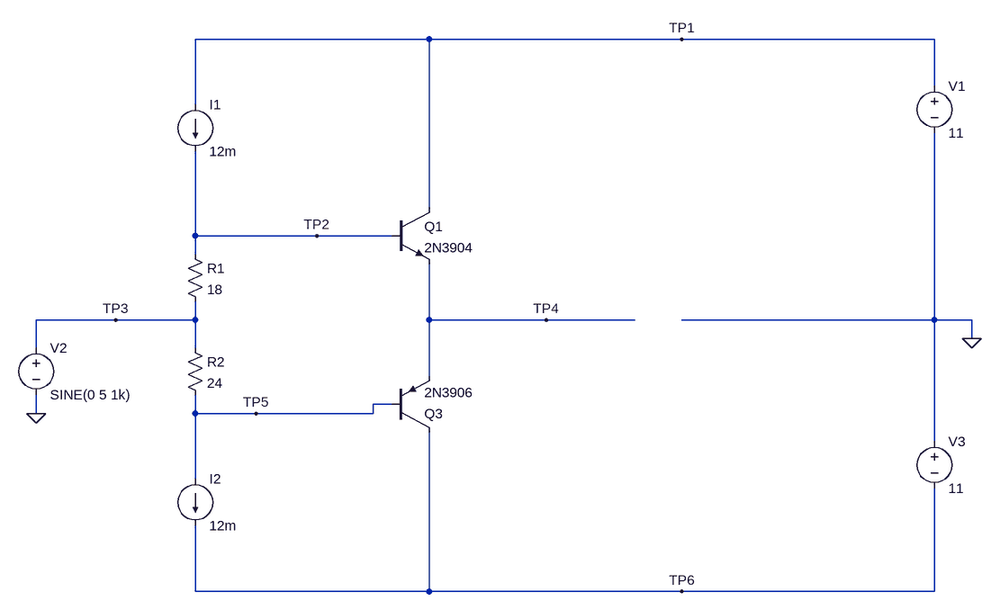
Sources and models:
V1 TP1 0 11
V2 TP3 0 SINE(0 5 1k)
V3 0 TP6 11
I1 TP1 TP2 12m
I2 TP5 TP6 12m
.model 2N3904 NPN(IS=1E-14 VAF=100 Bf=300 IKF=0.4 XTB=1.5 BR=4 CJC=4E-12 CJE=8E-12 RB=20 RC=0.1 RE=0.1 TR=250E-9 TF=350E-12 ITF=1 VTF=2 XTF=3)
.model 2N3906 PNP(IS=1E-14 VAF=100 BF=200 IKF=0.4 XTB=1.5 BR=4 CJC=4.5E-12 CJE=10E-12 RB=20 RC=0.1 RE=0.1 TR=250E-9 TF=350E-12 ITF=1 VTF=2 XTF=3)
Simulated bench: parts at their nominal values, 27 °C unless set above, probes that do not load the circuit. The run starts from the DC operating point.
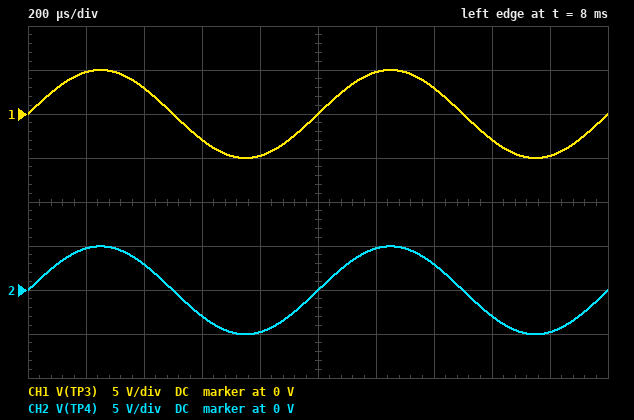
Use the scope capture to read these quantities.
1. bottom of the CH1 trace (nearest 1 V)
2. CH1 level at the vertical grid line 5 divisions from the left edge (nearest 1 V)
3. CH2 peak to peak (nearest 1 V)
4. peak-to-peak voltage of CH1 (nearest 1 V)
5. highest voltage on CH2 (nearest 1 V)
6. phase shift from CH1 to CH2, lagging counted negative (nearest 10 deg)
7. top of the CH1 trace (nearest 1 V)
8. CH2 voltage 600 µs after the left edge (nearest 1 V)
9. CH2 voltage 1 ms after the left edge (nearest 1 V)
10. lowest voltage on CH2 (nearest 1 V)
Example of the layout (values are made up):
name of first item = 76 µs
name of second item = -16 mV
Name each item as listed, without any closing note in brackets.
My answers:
bottom of the CH1 trace = -5 V
CH1 level at the vertical grid line 5 divisions from the left edge = 0 V
CH2 peak to peak = 10 V
peak-to-peak voltage of CH1 = 10 V
highest voltage on CH2 = 5 V
phase shift from CH1 to CH2, lagging counted negative = 0 deg
top of the CH1 trace = 5 V
CH2 voltage 600 µs after the left edge = -3 V
CH2 voltage 1 ms after the left edge = 0 V
lowest voltage on CH2 = -5 V
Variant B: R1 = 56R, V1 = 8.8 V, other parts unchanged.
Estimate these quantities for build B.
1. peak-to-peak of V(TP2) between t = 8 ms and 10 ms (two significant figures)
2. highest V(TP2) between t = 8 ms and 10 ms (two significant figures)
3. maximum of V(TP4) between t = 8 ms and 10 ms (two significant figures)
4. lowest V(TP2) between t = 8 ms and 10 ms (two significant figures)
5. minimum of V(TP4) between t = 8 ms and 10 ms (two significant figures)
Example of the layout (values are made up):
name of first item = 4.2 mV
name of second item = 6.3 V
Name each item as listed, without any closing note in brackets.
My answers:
peak-to-peak of V(TP2) between t = 8 ms and 10 ms = 10 V
highest V(TP2) between t = 8 ms and 10 ms = 5.7 V
maximum of V(TP4) between t = 8 ms and 10 ms = 5.2 V
lowest V(TP2) between t = 8 ms and 10 ms = -4.3 V
minimum of V(TP4) between t = 8 ms and 10 ms = -4.8 V
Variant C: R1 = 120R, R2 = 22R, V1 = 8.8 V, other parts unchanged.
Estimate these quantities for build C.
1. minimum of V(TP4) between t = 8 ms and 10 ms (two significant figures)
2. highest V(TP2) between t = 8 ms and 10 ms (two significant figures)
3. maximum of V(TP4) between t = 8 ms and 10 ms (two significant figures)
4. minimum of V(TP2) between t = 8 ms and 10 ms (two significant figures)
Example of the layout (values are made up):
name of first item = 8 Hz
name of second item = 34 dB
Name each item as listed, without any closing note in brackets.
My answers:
minimum of V(TP4) between t = 8 ms and 10 ms = -4.4 V
highest V(TP2) between t = 8 ms and 10 ms = 6.4 V
maximum of V(TP4) between t = 8 ms and 10 ms = 5.6 V
minimum of V(TP2) between t = 8 ms and 10 ms = -3.6 V
